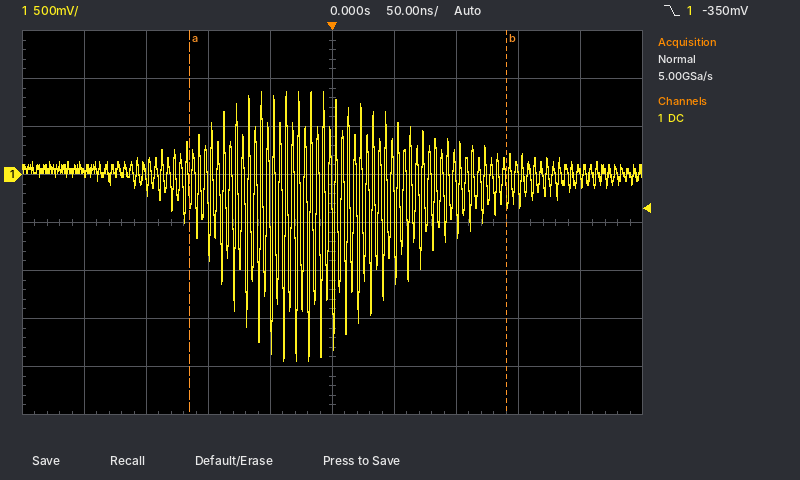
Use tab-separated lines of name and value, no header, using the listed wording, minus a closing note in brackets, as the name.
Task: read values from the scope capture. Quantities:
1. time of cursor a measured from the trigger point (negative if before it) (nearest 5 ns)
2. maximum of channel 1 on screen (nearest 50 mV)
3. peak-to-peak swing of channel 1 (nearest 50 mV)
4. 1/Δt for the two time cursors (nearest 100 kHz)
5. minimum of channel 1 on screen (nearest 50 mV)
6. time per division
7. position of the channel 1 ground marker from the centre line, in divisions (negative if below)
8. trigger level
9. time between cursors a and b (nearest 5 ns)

time of cursor a measured from the trigger point (negative if before it)	-115 ns
maximum of channel 1 on screen	850 mV
peak-to-peak swing of channel 1	2.80 V
1/Δt for the two time cursors	3.9 MHz
minimum of channel 1 on screen	-1.95 V
time per division	50 ns
position of the channel 1 ground marker from the centre line, in divisions	+1.0 div
trigger level	-350 mV
time between cursors a and b	255 ns
